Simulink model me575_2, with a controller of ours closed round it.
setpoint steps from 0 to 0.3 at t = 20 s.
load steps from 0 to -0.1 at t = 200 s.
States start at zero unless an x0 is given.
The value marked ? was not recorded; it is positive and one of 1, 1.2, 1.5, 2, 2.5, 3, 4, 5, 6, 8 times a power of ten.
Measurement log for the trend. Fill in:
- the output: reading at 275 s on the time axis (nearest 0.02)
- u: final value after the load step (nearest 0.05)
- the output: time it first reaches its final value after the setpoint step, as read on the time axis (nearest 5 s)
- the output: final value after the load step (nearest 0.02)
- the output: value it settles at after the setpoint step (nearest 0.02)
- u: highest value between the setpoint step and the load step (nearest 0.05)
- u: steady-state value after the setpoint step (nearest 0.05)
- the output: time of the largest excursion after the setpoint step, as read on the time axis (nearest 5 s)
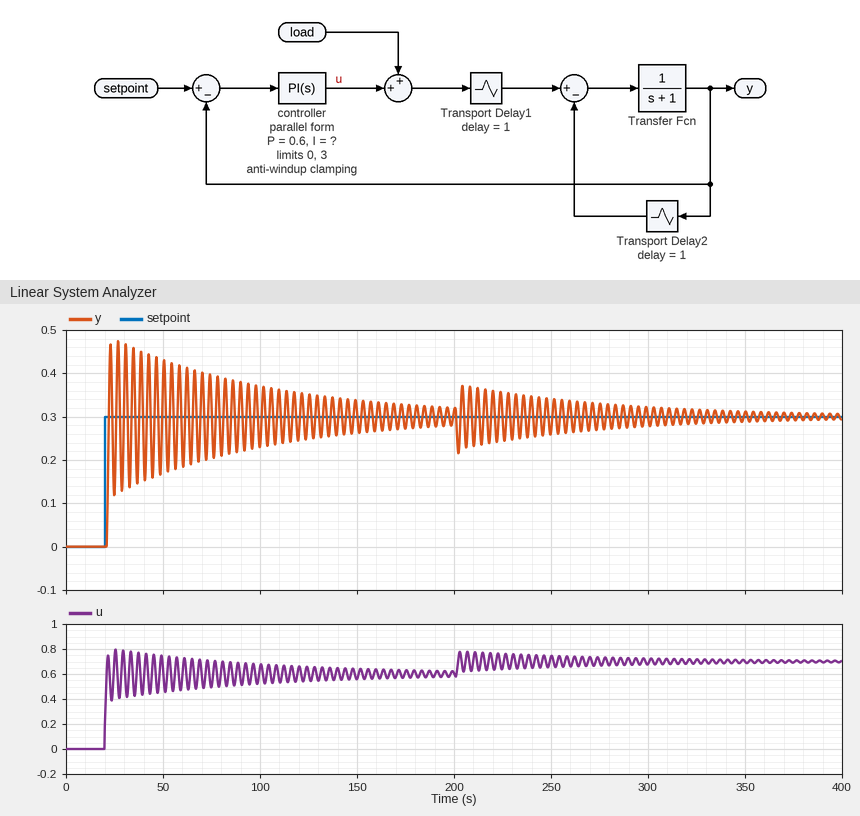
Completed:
0.32
0.70
20 s
0.30
0.30
0.80
0.60
25 s
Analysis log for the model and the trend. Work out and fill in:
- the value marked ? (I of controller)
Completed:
1.5
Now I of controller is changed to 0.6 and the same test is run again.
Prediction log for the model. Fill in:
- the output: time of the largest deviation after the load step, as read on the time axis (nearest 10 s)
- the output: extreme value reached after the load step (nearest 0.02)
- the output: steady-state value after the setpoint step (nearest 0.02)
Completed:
200 s
0.24
0.30
